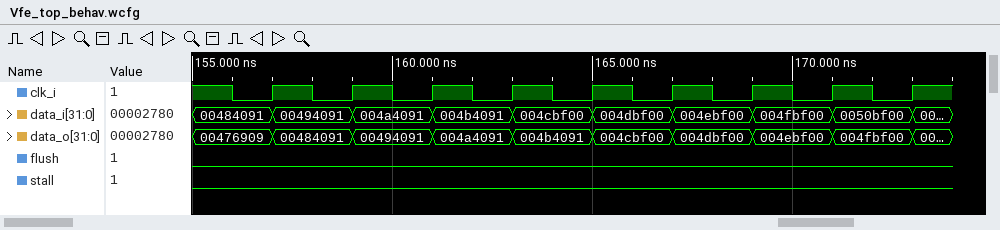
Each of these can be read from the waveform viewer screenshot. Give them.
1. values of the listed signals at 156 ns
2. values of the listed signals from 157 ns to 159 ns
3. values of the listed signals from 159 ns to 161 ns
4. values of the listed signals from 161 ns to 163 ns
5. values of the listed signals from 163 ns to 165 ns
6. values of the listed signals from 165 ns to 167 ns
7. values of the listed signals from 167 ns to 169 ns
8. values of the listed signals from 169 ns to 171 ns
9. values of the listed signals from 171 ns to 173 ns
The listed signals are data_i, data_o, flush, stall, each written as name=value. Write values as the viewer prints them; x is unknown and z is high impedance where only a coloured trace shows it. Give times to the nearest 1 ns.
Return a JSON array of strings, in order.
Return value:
["data_i=00484091, data_o=00476909, flush=0, stall=0", "data_i=00494091, data_o=00484091, flush=0, stall=0", "data_i=004a4091, data_o=00494091, flush=0, stall=0", "data_i=004b4091, data_o=004a4091, flush=0, stall=0", "data_i=004cbf00, data_o=004b4091, flush=0, stall=0", "data_i=004dbf00, data_o=004cbf00, flush=0, stall=0", "data_i=004ebf00, data_o=004dbf00, flush=0, stall=0", "data_i=004fbf00, data_o=004ebf00, flush=0, stall=0", "data_i=0050bf00, data_o=004fbf00, flush=0, stall=0"]
